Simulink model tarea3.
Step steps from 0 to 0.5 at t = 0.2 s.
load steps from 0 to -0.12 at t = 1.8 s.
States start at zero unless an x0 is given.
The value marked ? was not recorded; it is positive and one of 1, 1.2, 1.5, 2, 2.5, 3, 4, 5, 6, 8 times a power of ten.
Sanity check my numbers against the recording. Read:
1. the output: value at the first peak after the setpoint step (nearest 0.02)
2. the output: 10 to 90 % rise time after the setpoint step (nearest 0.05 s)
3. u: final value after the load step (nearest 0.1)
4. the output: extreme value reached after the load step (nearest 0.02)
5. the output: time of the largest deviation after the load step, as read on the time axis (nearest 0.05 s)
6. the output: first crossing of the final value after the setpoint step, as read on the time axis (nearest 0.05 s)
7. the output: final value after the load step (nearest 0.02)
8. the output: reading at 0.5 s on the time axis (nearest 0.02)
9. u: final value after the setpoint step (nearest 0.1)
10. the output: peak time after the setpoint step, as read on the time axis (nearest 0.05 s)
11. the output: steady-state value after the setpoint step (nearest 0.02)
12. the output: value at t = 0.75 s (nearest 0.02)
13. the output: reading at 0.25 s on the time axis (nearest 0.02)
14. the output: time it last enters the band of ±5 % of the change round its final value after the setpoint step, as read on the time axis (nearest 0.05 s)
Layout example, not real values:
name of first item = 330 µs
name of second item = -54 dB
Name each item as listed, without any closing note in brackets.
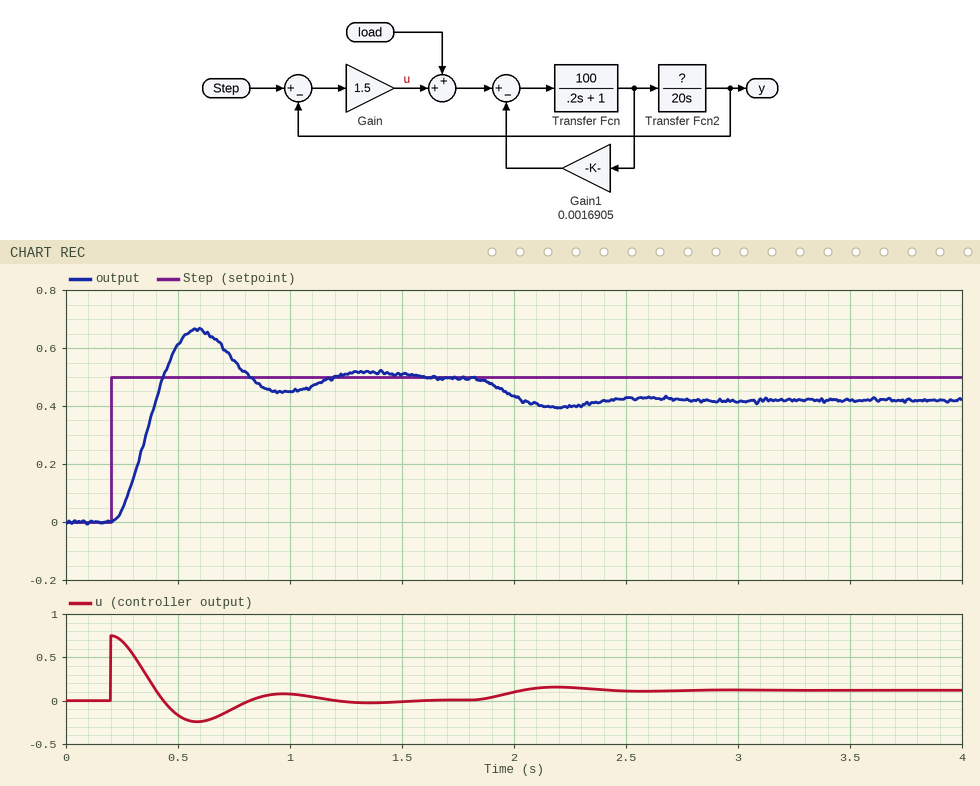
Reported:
the output: value at the first peak after the setpoint step = 0.66
the output: 10 to 90 % rise time after the setpoint step = 0.15 s
u: final value after the load step = 0.1
the output: extreme value reached after the load step = 0.40
the output: time of the largest deviation after the load step, as read on the time axis = 2.20 s
the output: first crossing of the final value after the setpoint step, as read on the time axis = 0.45 s
the output: final value after the load step = 0.42
the output: reading at 0.5 s on the time axis = 0.62
u: final value after the setpoint step = 0.0
the output: peak time after the setpoint step, as read on the time axis = 0.60 s
the output: steady-state value after the setpoint step = 0.50
the output: value at t = 0.75 s = 0.56
the output: reading at 0.25 s on the time axis = 0.04
the output: time it last enters the band of ±5 % of the change round its final value after the setpoint step, as read on the time axis = 1.10 s
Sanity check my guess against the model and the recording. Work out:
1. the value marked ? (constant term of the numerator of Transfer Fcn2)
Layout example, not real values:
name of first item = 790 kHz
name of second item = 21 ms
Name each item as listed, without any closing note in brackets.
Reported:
the value marked ? = 2
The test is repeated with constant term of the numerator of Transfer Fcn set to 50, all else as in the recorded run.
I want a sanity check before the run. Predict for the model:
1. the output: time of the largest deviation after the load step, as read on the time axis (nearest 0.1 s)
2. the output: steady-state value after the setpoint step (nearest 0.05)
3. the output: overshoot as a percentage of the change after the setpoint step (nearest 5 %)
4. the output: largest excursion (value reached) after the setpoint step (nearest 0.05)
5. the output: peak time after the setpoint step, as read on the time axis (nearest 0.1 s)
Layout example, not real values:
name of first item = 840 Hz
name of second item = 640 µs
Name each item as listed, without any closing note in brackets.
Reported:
the output: time of the largest deviation after the load step, as read on the time axis = 2.4 s
the output: steady-state value after the setpoint step = 0.50
the output: overshoot as a percentage of the change after the setpoint step = 20 %
the output: largest excursion (value reached) after the setpoint step = 0.60
the output: peak time after the setpoint step, as read on the time axis = 0.8 s
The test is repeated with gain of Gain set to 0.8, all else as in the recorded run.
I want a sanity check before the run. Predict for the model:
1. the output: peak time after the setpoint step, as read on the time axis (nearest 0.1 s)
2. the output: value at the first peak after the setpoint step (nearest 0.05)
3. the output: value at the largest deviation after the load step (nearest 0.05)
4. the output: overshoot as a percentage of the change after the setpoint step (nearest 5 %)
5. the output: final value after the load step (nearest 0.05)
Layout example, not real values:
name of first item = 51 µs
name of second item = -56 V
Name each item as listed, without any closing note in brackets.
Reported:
the output: peak time after the setpoint step, as read on the time axis = 0.8 s
the output: value at the first peak after the setpoint step = 0.60
the output: value at the largest deviation after the load step = 0.30
the output: overshoot as a percentage of the change after the setpoint step = 20 %
the output: final value after the load step = 0.35
